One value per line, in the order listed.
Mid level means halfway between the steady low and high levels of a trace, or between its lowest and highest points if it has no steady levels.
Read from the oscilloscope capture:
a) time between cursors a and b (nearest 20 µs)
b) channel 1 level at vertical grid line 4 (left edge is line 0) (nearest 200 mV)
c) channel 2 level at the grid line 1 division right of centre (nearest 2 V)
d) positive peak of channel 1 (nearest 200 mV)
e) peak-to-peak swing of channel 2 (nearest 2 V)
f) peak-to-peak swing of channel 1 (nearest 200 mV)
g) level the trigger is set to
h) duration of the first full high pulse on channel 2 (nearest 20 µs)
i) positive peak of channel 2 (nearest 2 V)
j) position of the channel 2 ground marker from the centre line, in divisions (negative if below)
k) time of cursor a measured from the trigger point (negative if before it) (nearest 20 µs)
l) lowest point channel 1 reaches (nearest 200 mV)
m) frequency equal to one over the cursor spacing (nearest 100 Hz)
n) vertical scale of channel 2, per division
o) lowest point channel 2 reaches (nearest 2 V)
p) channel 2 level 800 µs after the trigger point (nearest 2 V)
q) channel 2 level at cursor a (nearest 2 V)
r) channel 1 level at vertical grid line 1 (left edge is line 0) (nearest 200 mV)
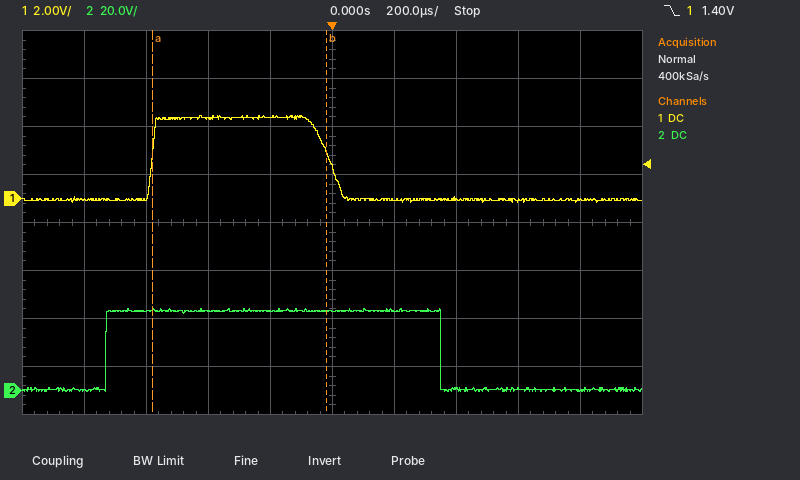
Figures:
560 µs
3.4 V
34 V
3.4 V
34 V
3.6 V
1.40 V
1.08 ms
34 V
-3.5 div
-580 µs
-200 mV
1.8 kHz
20 V
0 V
0 V
34 V
0.0 V
